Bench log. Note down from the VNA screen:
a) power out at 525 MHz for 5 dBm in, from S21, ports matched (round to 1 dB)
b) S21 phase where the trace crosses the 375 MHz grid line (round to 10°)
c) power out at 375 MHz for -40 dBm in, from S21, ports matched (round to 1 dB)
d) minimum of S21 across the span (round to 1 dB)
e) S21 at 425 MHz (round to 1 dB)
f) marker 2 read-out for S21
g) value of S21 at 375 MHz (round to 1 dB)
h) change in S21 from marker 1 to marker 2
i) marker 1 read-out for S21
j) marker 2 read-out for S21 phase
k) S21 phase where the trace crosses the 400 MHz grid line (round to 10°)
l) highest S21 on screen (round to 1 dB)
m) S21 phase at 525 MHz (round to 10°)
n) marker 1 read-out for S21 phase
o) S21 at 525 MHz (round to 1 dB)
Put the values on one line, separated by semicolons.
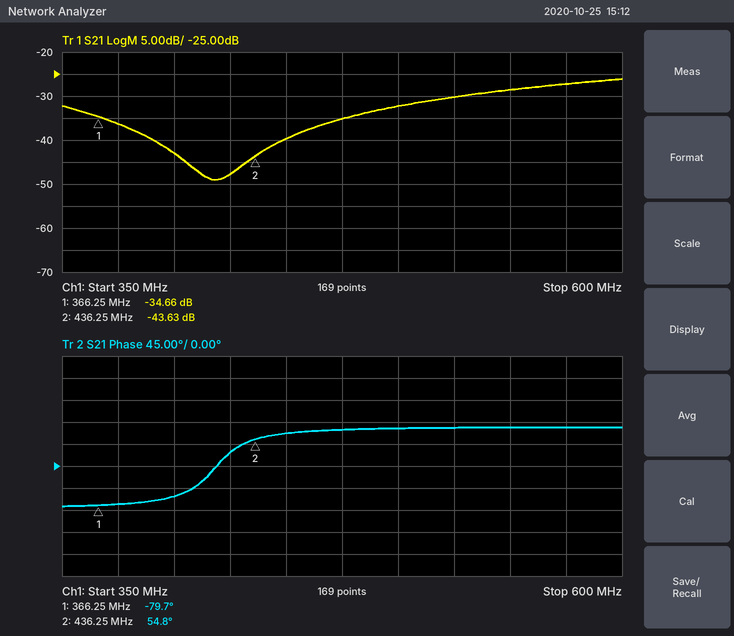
-25 dBm; -80°; -76 dBm; -49 dB; -48 dB; -43.63 dB; -36 dB; -8.97 dB; -34.66 dB; 54.8°; -60°; -26 dB; 80°; -79.7°; -30 dB
